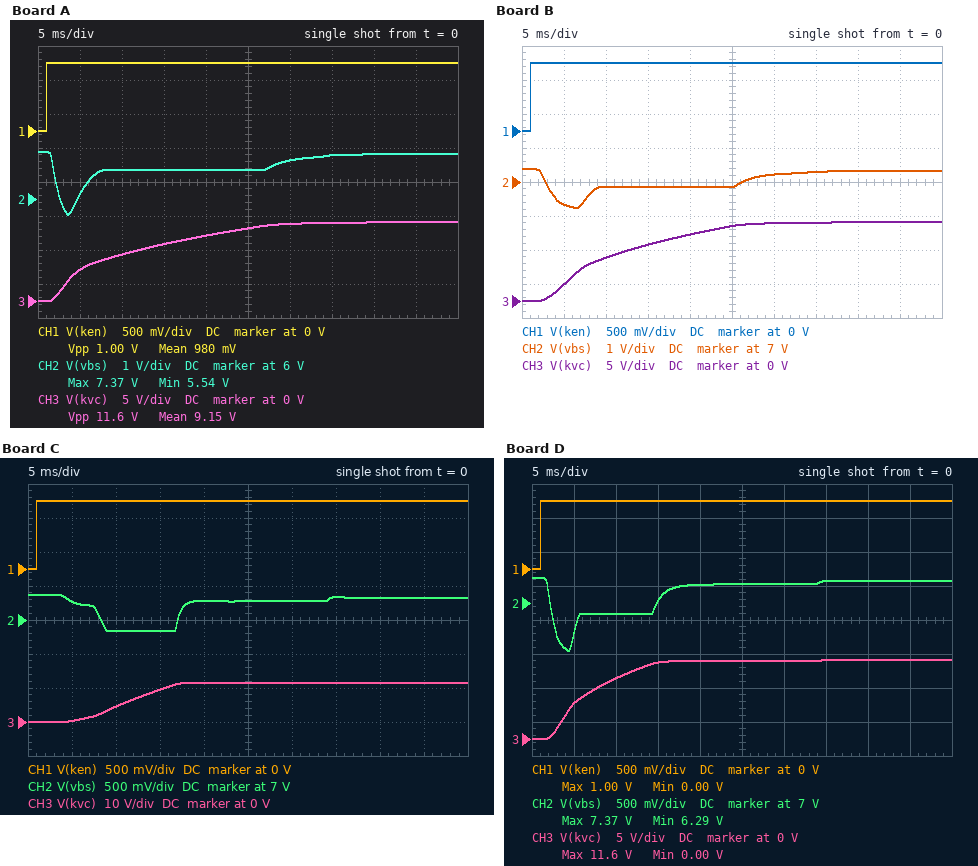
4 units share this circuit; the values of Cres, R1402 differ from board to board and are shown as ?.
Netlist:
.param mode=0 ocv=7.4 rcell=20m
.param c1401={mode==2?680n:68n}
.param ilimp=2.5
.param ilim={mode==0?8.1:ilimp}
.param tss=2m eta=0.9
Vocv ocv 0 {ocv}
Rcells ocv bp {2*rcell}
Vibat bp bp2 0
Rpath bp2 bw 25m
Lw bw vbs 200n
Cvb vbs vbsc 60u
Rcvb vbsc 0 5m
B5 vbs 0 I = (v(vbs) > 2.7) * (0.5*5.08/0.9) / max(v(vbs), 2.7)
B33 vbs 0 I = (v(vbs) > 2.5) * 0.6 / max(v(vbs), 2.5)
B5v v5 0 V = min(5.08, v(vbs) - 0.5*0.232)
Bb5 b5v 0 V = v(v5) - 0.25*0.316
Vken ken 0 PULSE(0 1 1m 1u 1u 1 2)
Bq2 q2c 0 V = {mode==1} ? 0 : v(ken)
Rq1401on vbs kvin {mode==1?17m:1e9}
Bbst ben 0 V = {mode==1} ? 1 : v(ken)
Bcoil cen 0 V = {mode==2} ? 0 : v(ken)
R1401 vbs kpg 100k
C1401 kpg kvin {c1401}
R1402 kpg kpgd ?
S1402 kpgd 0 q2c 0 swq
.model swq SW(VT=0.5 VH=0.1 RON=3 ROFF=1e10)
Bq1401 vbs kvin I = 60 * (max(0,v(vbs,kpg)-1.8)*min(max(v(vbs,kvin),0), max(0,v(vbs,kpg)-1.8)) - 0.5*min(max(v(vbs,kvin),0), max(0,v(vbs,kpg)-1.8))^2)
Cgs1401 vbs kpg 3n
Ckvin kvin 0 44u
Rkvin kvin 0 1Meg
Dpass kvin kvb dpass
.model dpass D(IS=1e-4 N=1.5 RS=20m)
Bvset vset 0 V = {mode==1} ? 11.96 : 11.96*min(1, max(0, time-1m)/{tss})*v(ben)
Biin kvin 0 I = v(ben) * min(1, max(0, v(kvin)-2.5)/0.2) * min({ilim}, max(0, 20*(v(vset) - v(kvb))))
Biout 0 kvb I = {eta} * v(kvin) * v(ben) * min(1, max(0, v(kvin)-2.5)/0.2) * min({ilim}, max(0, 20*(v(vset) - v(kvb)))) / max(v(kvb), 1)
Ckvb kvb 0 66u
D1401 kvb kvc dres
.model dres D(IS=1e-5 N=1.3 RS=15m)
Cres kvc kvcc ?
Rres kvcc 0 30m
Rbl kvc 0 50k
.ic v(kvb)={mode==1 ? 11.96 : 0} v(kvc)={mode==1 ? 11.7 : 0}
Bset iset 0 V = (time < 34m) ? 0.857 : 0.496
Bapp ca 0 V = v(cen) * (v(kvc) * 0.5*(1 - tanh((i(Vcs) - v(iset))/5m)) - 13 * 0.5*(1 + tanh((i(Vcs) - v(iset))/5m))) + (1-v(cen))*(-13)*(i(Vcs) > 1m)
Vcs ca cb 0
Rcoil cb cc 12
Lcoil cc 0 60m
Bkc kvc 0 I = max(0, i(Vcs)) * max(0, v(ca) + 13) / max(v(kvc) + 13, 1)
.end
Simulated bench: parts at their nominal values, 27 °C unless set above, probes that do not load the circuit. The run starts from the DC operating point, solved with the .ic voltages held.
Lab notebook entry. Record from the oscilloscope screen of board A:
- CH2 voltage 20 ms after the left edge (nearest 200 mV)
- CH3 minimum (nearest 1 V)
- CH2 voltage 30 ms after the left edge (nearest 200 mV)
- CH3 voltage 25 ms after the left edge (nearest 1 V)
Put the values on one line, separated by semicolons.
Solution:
6.8 V; 0 V; 7.2 V; 11 V
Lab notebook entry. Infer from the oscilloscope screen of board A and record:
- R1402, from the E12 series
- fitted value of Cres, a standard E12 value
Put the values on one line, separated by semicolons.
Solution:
15 kΩ; 18 mF
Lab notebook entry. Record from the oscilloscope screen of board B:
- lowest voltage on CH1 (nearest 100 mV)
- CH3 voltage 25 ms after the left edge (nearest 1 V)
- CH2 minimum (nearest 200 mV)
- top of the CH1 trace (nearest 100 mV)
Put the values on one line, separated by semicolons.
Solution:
0 V; 11 V; 6.2 V; 1.0 V
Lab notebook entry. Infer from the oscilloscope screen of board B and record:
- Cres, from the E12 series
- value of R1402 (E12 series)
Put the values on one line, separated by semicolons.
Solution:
15 mF; 33 kΩ
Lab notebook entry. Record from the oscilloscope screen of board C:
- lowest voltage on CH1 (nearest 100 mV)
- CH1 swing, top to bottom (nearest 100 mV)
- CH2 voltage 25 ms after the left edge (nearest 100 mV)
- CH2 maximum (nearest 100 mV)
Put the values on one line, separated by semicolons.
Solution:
0 V; 1.0 V; 7.3 V; 7.4 V
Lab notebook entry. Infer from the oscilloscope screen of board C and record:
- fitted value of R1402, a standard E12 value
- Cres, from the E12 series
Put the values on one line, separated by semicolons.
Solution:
82 kΩ; 3.9 mF
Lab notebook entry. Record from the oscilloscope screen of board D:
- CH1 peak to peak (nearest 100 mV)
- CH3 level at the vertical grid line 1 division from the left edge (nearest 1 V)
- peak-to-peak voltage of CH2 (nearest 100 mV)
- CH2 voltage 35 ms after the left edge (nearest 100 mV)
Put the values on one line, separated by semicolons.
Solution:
1.0 V; 5 V; 1.1 V; 7.3 V
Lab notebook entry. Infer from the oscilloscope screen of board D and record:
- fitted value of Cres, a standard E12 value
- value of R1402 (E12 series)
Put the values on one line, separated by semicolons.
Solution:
8.2 mF; 22 kΩ
